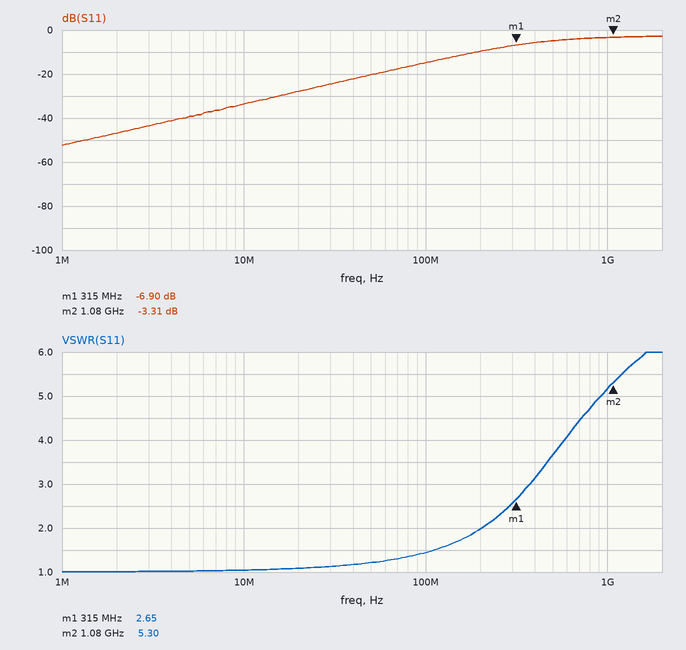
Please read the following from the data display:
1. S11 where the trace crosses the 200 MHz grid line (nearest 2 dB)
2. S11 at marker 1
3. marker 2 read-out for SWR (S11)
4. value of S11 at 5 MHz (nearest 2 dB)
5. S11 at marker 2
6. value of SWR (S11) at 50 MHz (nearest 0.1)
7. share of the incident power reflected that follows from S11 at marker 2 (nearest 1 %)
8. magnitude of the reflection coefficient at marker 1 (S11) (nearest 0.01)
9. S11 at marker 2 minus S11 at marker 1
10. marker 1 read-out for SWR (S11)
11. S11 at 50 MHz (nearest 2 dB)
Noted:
-10 dB
-6.90 dB
5.30
-40 dB
-3.31 dB
1.2
47 %
0.45
3.59 dB
2.65
-20 dB
